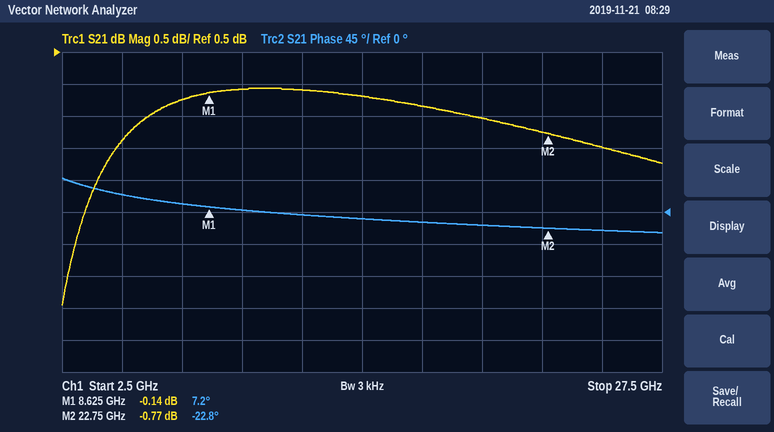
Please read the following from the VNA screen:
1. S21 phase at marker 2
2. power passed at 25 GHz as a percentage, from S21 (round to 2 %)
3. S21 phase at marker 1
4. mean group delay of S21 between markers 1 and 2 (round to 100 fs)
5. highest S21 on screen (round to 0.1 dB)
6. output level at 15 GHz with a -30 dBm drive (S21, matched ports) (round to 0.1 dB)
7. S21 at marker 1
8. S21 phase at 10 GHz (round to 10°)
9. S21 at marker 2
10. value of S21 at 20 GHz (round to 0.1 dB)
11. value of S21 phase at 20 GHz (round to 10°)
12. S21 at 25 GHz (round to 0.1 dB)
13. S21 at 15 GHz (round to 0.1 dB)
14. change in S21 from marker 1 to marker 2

-22.8°
80 %
7.2°
5.9 ps
-0.1 dB
-30.2 dBm
-0.14 dB
0°
-0.77 dB
-0.5 dB
-20°
-1.0 dB
-0.2 dB
-0.63 dB
